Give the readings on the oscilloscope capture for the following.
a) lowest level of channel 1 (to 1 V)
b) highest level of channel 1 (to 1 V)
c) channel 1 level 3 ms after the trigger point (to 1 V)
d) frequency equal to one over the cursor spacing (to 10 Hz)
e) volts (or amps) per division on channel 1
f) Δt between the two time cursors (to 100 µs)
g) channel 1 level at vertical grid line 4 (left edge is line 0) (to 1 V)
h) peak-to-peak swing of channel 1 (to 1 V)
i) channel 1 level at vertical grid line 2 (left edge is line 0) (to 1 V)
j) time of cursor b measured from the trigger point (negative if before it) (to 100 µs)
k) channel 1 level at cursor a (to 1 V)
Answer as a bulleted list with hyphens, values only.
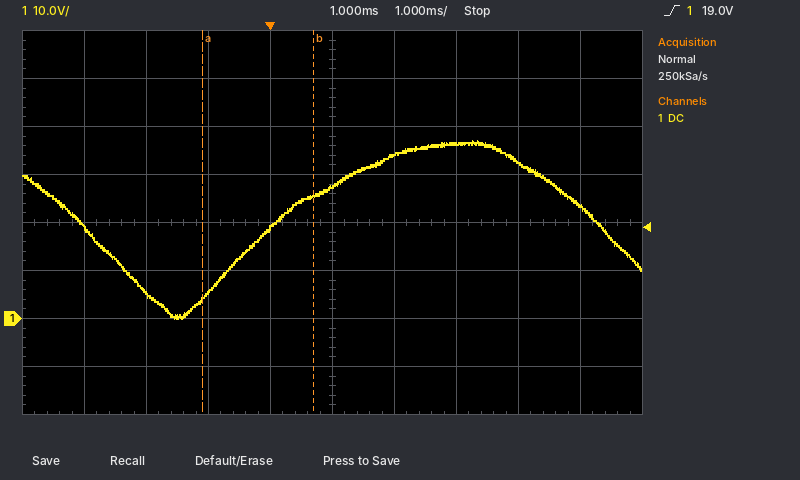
- 0 V
- 37 V
- 36 V
- 560 Hz
- 10 V
- 1.8 ms
- 19 V
- 37 V
- 5 V
- +700 µs
- 4 V
